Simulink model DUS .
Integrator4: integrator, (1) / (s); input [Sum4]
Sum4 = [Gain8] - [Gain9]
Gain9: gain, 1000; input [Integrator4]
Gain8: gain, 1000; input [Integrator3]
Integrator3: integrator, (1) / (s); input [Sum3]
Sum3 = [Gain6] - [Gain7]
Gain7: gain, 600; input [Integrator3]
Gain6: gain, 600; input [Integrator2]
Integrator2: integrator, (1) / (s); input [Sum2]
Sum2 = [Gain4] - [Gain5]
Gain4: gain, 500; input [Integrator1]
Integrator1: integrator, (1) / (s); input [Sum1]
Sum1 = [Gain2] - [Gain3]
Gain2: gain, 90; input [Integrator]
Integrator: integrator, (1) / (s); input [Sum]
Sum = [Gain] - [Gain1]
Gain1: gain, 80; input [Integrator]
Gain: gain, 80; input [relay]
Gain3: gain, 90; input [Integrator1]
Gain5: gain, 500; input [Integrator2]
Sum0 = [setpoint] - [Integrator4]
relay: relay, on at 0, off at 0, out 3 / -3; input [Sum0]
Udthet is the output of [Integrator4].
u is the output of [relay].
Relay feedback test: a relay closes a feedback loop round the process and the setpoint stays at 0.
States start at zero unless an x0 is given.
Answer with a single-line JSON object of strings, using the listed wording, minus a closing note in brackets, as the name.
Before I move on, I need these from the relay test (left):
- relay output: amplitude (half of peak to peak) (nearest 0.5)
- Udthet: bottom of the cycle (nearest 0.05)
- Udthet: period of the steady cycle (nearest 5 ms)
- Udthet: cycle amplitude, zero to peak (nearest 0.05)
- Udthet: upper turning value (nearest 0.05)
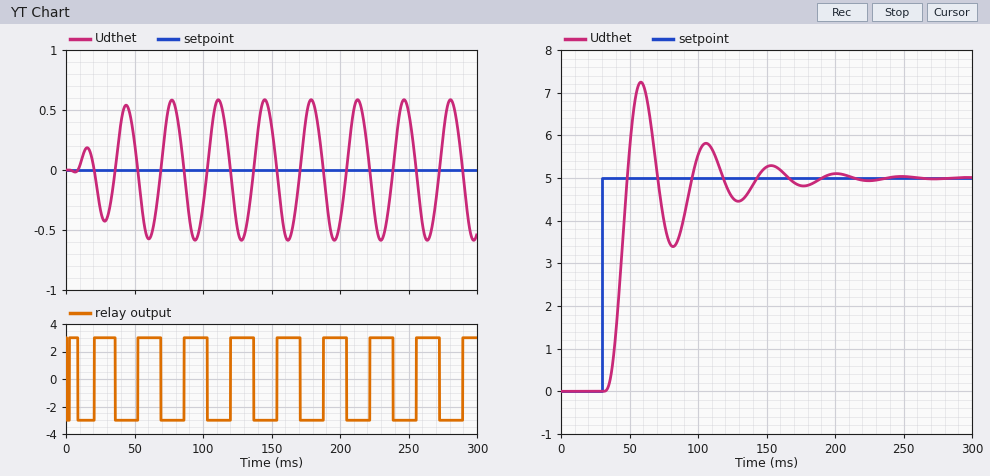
{"relay output: amplitude (half of peak to peak)": "3.0", "Udthet: bottom of the cycle": "-0.60", "Udthet: period of the steady cycle": "35 ms", "Udthet: cycle amplitude, zero to peak": "0.60", "Udthet: upper turning value": "0.60"}
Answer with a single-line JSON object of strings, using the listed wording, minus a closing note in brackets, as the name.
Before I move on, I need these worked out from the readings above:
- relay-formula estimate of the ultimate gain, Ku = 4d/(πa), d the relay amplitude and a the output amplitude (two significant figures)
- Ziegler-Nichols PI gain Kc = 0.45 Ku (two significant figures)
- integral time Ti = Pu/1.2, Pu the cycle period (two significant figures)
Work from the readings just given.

{"relay-formula estimate of the ultimate gain, Ku = 4d/(πa), d the relay amplitude and a the output amplitude": "6.4", "Ziegler-Nichols PI gain Kc = 0.45 Ku": "2.9", "integral time Ti = Pu/1.2, Pu the cycle period": "29 ms"}
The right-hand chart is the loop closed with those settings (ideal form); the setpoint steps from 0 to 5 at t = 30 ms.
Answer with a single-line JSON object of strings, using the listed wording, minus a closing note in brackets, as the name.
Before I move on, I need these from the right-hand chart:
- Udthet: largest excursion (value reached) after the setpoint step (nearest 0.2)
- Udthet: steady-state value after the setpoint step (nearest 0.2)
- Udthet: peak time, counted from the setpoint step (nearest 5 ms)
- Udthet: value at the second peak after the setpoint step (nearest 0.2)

{"Udthet: largest excursion (value reached) after the setpoint step": "7.2", "Udthet: steady-state value after the setpoint step": "5.0", "Udthet: peak time, counted from the setpoint step": "30 ms", "Udthet: value at the second peak after the setpoint step": "5.8"}
